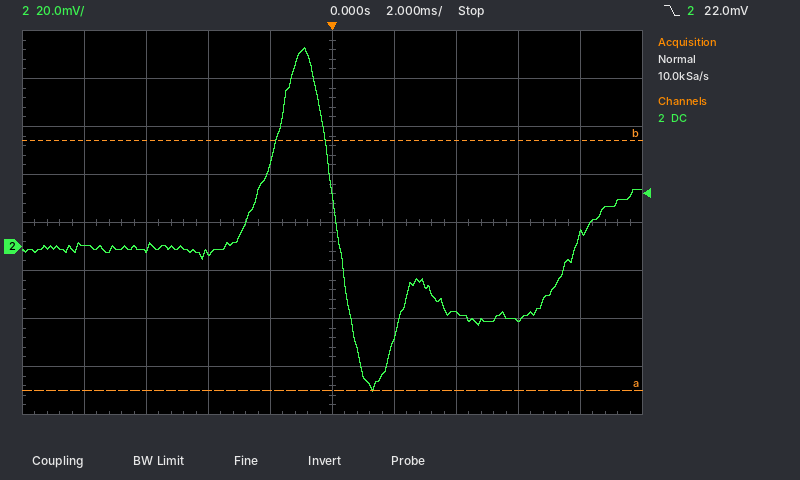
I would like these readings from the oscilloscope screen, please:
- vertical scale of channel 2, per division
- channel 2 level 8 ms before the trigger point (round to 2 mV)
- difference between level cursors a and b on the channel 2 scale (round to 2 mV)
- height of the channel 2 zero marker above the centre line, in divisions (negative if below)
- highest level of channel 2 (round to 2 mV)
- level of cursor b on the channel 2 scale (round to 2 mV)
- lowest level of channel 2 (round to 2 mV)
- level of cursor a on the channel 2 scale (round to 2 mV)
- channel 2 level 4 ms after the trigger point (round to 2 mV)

20 mV
0 mV
104 mV
-0.5 div
82 mV
44 mV
-60 mV
-60 mV
-28 mV
